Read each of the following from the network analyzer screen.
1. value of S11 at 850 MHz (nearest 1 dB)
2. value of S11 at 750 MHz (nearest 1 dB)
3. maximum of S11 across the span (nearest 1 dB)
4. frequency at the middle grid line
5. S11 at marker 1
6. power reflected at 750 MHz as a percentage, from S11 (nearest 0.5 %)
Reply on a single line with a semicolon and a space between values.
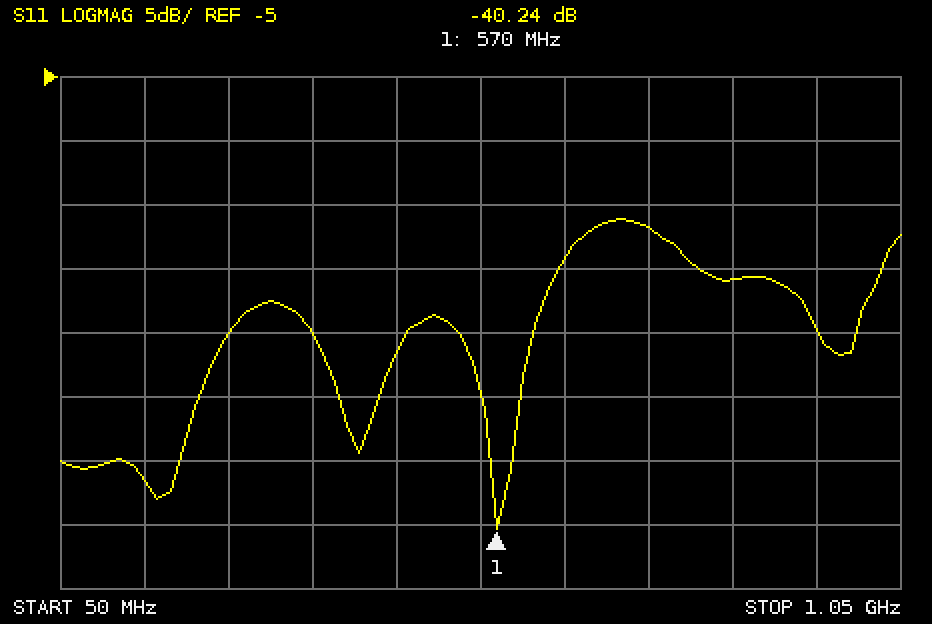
-21 dB; -17 dB; -16 dB; 550 MHz; -40.24 dB; 2.0 %
